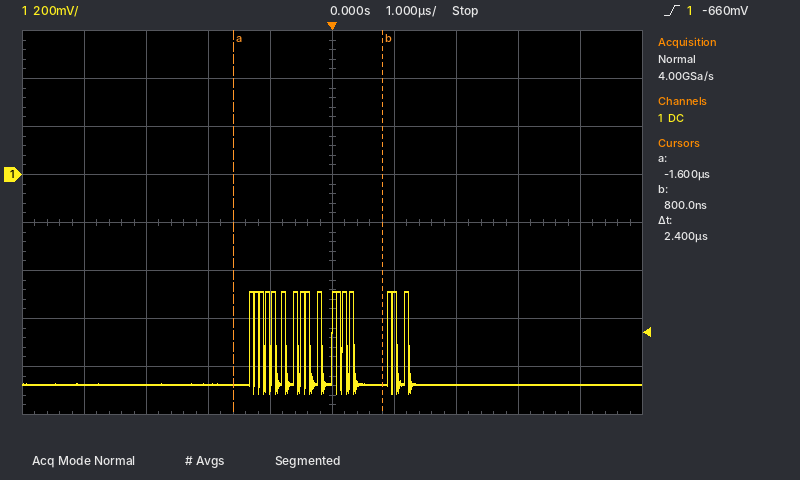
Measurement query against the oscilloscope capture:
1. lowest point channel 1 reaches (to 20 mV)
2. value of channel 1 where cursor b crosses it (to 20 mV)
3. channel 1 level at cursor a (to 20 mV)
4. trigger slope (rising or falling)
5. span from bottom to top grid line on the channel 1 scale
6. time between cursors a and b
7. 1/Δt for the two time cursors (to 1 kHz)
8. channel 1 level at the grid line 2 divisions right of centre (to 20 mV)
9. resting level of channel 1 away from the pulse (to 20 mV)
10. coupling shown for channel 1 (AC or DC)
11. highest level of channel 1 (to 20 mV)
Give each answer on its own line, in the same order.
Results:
-920 mV
-880 mV
-880 mV
rising
1.6 V
2.4 µs
417 kHz
-880 mV
-880 mV
DC
-480 mV
